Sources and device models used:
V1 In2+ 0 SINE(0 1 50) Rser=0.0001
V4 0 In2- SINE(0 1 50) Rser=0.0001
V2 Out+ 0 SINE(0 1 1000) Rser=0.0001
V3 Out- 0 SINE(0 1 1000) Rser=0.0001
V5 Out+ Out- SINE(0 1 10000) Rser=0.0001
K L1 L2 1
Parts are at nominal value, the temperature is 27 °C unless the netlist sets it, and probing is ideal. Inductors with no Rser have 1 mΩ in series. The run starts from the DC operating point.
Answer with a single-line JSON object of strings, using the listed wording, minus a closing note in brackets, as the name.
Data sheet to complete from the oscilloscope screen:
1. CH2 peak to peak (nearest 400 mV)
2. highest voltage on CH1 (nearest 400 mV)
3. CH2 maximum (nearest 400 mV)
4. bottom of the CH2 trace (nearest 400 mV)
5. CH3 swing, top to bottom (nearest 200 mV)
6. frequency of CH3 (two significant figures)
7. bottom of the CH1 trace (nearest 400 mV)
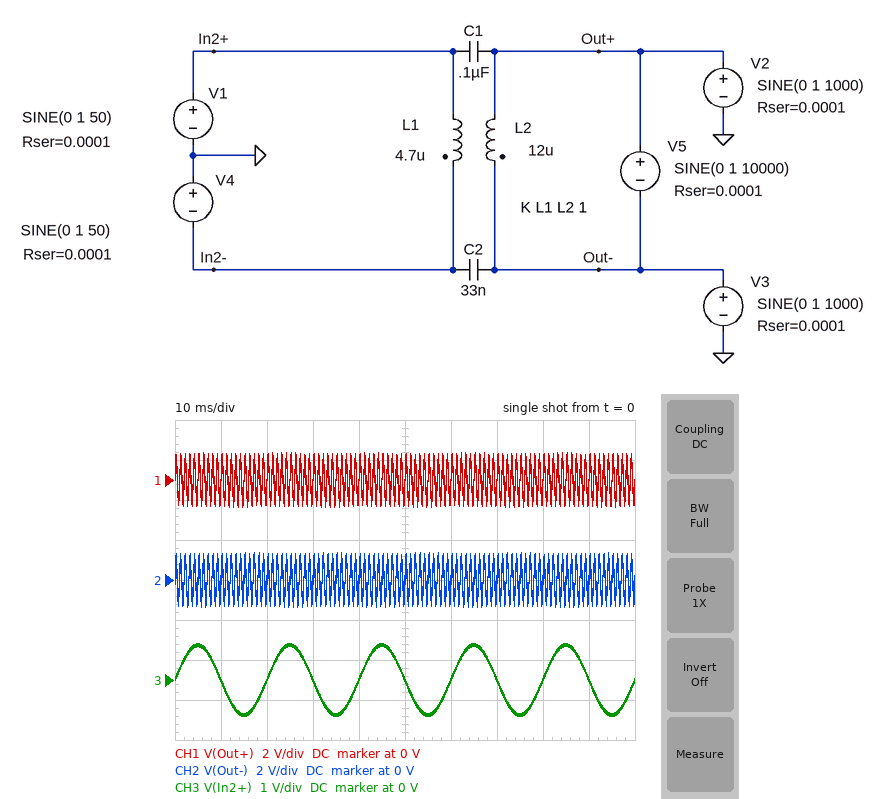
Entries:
{"CH2 peak to peak": "2.8 V", "highest voltage on CH1": "1.2 V", "CH2 maximum": "1.2 V", "bottom of the CH2 trace": "-1.2 V", "CH3 swing, top to bottom": "1.8 V", "frequency of CH3": "50 Hz", "bottom of the CH1 trace": "-1.2 V"}
